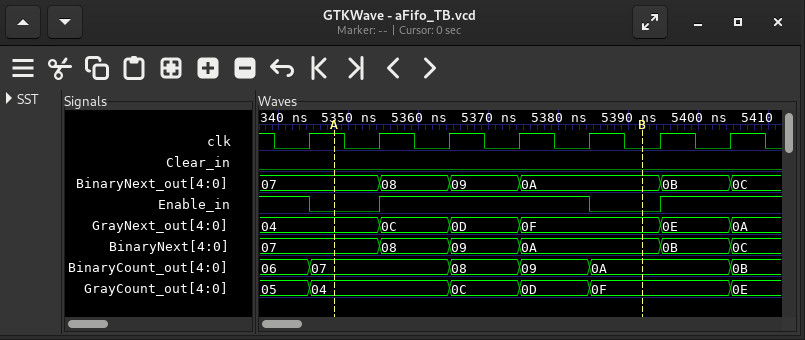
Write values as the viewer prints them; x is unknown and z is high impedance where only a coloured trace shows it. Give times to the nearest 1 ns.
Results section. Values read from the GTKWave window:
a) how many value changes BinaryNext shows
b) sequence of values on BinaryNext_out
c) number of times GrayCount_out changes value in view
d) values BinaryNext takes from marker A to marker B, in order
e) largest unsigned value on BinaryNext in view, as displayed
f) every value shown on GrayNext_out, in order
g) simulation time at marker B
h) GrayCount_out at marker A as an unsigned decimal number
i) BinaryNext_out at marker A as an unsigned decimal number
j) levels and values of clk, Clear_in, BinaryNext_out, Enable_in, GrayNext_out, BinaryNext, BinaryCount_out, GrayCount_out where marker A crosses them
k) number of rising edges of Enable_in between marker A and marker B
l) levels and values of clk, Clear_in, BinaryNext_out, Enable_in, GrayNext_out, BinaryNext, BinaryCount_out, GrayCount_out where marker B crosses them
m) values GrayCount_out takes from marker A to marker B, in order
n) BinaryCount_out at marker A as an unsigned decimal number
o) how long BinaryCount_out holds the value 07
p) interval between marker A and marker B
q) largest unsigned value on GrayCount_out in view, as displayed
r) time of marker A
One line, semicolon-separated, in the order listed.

5; 07, 08, 09, 0A, 0B, 0C; 5; 07, 08, 09, 0A; 0C; 04, 0C, 0D, 0F, 0E, 0A; 5392 ns; 4; 7; clk=1, Clear_in=0, BinaryNext_out=07, Enable_in=0, GrayNext_out=04, BinaryNext=07, BinaryCount_out=07, GrayCount_out=04; 1; clk=0, Clear_in=0, BinaryNext_out=0A, Enable_in=0, GrayNext_out=0F, BinaryNext=0A, BinaryCount_out=0A, GrayCount_out=0F; 04, 0C, 0D, 0F; 7; 20 ns; 44 ns; 0F; 5348 ns
